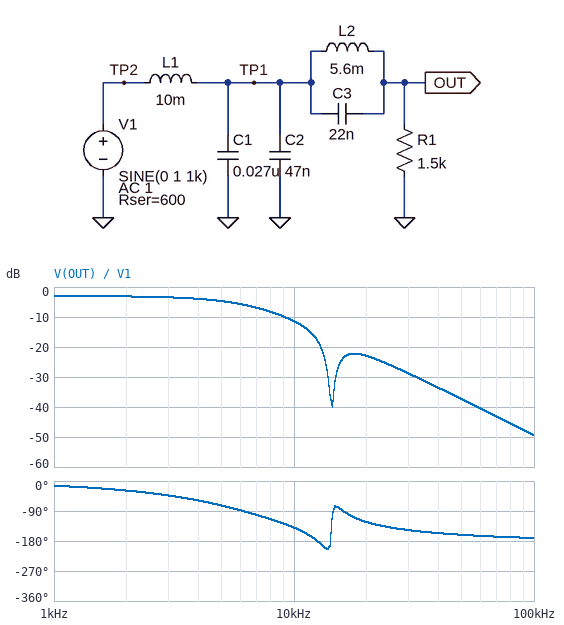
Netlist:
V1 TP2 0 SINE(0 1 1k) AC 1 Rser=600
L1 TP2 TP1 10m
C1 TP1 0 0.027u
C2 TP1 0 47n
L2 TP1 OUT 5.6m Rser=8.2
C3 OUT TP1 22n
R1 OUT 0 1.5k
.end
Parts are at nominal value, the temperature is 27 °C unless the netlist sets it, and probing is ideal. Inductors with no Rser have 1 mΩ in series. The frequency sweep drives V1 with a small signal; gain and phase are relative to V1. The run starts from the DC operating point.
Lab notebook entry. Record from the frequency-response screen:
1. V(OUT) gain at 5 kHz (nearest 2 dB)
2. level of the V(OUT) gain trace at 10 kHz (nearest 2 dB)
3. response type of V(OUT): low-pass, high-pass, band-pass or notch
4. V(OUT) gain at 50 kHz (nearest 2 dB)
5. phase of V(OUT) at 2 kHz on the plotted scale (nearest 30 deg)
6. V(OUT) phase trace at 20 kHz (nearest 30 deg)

-4 dB
-12 dB
low-pass
-38 dB
-30 deg
-120 deg
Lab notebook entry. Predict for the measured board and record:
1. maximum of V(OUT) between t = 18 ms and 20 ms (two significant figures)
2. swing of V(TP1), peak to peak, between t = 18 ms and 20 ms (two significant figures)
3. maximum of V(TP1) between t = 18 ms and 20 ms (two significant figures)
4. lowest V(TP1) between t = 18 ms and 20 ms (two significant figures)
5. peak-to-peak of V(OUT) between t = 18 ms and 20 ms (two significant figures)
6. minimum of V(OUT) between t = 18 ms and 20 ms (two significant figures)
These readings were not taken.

710 mV
1.4 V
710 mV
-710 mV
1.4 V
-710 mV
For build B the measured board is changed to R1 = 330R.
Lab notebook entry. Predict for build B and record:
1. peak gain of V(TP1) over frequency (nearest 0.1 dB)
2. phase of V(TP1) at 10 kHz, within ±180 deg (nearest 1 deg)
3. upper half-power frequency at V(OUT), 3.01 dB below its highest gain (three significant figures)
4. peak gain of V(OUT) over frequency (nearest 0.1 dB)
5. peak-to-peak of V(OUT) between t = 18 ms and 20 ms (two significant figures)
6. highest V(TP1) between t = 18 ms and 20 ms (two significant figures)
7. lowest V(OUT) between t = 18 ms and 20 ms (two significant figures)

-6.3 dB
-109 deg
8.81 kHz
-9.1 dB
700 mV
360 mV
-350 mV
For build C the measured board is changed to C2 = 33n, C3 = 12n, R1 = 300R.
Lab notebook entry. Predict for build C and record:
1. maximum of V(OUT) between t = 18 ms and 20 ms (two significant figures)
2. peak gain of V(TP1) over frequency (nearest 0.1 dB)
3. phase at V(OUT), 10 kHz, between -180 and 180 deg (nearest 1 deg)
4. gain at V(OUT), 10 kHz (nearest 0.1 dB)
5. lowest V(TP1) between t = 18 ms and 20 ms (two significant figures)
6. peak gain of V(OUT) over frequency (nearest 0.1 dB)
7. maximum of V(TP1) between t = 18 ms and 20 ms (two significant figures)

330 mV
-5.6 dB
-143 deg
-11.6 dB
-340 mV
-9.5 dB
340 mV
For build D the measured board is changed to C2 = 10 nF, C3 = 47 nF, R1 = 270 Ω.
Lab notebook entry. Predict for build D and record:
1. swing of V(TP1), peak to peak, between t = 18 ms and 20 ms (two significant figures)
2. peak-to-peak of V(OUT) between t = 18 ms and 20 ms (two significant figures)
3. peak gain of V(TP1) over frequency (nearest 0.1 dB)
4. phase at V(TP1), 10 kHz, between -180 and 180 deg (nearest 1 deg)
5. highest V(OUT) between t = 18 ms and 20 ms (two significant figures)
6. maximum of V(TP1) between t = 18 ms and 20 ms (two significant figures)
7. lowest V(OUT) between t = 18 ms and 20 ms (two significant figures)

640 mV
610 mV
0 dB
-108 deg
310 mV
320 mV
-310 mV
